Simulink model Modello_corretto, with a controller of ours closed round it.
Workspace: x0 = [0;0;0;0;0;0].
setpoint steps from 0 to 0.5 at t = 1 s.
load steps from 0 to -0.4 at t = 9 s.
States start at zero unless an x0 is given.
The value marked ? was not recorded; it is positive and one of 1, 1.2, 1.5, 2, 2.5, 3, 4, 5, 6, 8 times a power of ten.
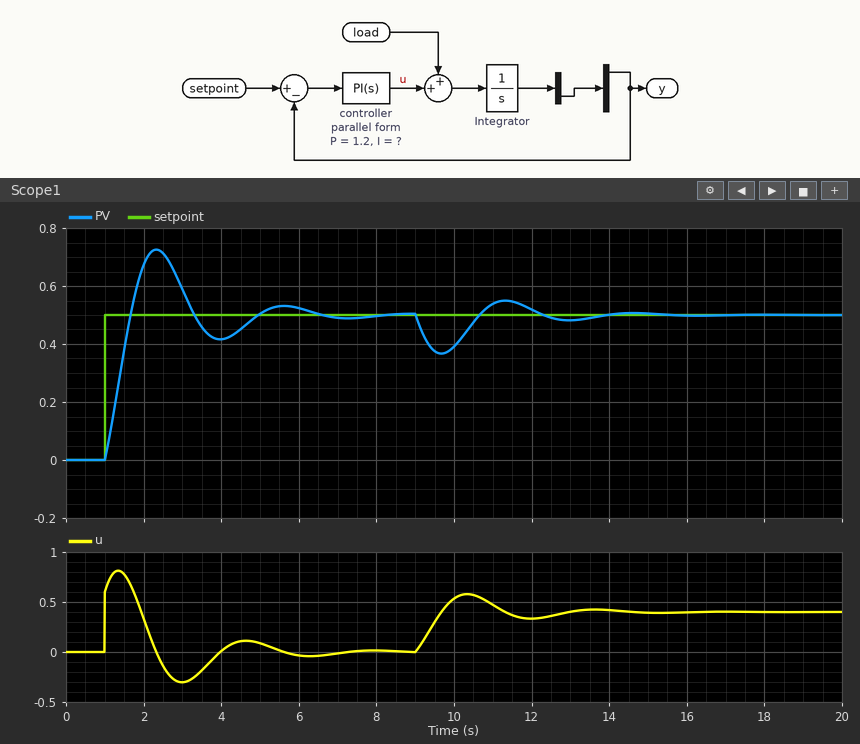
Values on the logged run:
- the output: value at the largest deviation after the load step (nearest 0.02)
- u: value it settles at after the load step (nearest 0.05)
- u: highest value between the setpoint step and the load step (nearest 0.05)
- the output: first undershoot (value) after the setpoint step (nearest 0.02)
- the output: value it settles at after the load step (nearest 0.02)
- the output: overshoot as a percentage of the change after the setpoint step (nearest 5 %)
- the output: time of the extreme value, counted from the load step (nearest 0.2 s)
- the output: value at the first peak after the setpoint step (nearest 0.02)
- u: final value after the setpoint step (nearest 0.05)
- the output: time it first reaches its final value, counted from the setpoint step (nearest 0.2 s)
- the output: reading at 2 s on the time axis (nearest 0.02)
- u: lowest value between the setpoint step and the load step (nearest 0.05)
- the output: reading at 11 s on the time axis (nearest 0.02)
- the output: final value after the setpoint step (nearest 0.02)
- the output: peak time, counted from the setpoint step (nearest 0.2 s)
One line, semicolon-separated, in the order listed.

0.36; 0.40; 0.80; 0.42; 0.50; 45 %; 0.6 s; 0.72; 0.00; 0.6 s; 0.68; -0.30; 0.54; 0.50; 1.4 s
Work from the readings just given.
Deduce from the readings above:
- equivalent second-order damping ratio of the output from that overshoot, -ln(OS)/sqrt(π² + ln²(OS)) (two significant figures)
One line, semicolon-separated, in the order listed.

0.25
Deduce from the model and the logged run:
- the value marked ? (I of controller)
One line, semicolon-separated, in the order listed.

4
